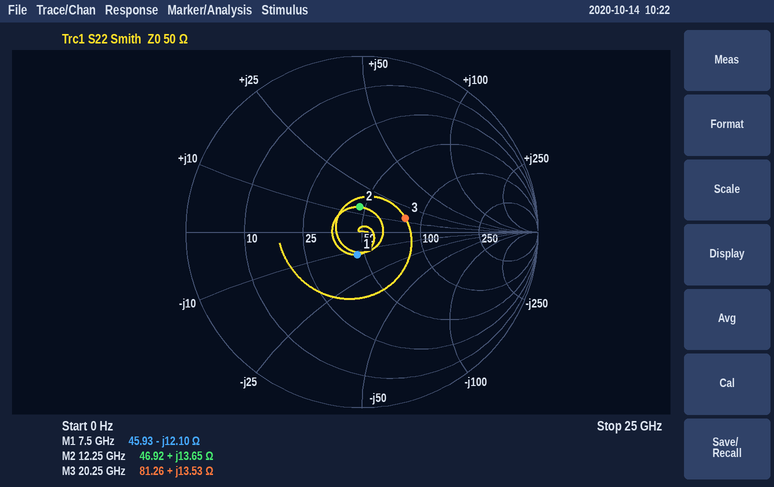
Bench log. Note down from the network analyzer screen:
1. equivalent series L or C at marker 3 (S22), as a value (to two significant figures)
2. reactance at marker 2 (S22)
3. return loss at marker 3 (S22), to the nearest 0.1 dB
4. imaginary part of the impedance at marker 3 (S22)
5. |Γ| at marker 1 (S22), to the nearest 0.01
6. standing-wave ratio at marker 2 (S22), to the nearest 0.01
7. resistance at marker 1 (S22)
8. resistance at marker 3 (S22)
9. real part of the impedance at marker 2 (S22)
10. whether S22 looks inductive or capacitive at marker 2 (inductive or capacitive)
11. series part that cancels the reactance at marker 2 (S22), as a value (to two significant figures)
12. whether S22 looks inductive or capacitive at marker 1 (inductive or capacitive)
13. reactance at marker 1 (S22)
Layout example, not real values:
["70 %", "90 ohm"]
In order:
["110 pH", "+13.65 Ω", "11.8 dB", "+13.53 Ω", "0.13", "1.33", "45.93 Ω", "81.26 Ω", "46.92 Ω", "inductive", "950 fF", "capacitive", "-12.10 Ω"]
